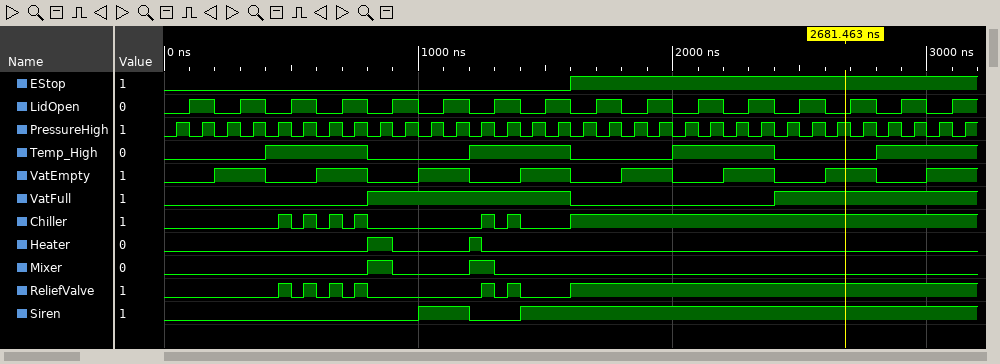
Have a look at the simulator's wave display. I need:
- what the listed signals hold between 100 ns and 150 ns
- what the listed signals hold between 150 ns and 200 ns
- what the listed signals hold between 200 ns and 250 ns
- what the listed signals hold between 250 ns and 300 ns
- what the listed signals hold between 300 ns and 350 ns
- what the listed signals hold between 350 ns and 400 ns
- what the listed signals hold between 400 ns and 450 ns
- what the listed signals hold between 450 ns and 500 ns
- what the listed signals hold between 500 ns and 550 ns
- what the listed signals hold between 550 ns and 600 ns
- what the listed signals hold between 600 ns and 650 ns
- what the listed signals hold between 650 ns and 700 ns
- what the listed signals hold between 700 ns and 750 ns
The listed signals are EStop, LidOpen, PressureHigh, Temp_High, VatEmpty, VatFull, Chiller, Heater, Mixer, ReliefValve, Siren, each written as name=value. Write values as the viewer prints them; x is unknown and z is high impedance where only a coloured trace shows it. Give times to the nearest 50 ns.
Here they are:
EStop=0, LidOpen=1, PressureHigh=0, Temp_High=0, VatEmpty=0, VatFull=0, Chiller=0, Heater=0, Mixer=0, ReliefValve=0, Siren=0
EStop=0, LidOpen=1, PressureHigh=1, Temp_High=0, VatEmpty=0, VatFull=0, Chiller=0, Heater=0, Mixer=0, ReliefValve=0, Siren=0
EStop=0, LidOpen=0, PressureHigh=0, Temp_High=0, VatEmpty=1, VatFull=0, Chiller=0, Heater=0, Mixer=0, ReliefValve=0, Siren=0
EStop=0, LidOpen=0, PressureHigh=1, Temp_High=0, VatEmpty=1, VatFull=0, Chiller=0, Heater=0, Mixer=0, ReliefValve=0, Siren=0
EStop=0, LidOpen=1, PressureHigh=0, Temp_High=0, VatEmpty=1, VatFull=0, Chiller=0, Heater=0, Mixer=0, ReliefValve=0, Siren=0
EStop=0, LidOpen=1, PressureHigh=1, Temp_High=0, VatEmpty=1, VatFull=0, Chiller=0, Heater=0, Mixer=0, ReliefValve=0, Siren=0
EStop=0, LidOpen=0, PressureHigh=0, Temp_High=1, VatEmpty=0, VatFull=0, Chiller=0, Heater=0, Mixer=0, ReliefValve=0, Siren=0
EStop=0, LidOpen=0, PressureHigh=1, Temp_High=1, VatEmpty=0, VatFull=0, Chiller=1, Heater=0, Mixer=0, ReliefValve=1, Siren=0
EStop=0, LidOpen=1, PressureHigh=0, Temp_High=1, VatEmpty=0, VatFull=0, Chiller=0, Heater=0, Mixer=0, ReliefValve=0, Siren=0
EStop=0, LidOpen=1, PressureHigh=1, Temp_High=1, VatEmpty=0, VatFull=0, Chiller=1, Heater=0, Mixer=0, ReliefValve=1, Siren=0
EStop=0, LidOpen=0, PressureHigh=0, Temp_High=1, VatEmpty=1, VatFull=0, Chiller=0, Heater=0, Mixer=0, ReliefValve=0, Siren=0
EStop=0, LidOpen=0, PressureHigh=1, Temp_High=1, VatEmpty=1, VatFull=0, Chiller=1, Heater=0, Mixer=0, ReliefValve=1, Siren=0
EStop=0, LidOpen=1, PressureHigh=0, Temp_High=1, VatEmpty=1, VatFull=0, Chiller=0, Heater=0, Mixer=0, ReliefValve=0, Siren=0
